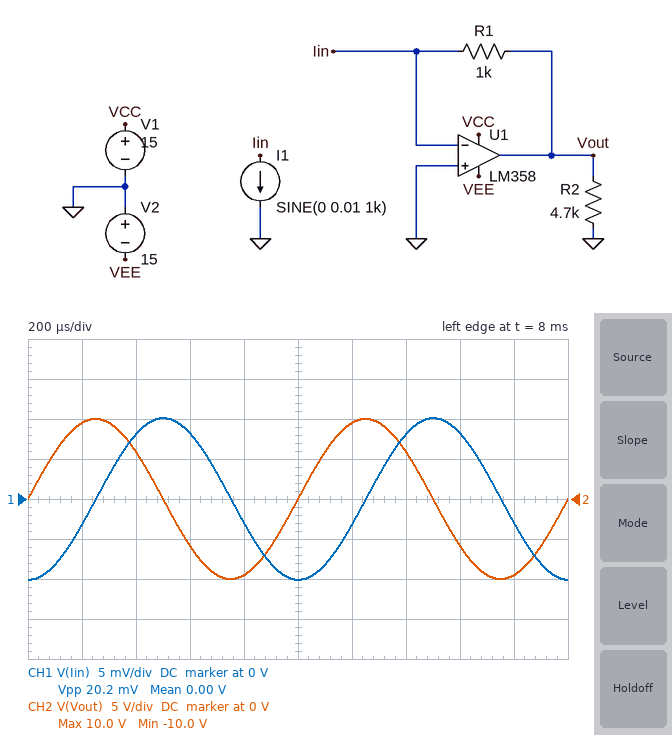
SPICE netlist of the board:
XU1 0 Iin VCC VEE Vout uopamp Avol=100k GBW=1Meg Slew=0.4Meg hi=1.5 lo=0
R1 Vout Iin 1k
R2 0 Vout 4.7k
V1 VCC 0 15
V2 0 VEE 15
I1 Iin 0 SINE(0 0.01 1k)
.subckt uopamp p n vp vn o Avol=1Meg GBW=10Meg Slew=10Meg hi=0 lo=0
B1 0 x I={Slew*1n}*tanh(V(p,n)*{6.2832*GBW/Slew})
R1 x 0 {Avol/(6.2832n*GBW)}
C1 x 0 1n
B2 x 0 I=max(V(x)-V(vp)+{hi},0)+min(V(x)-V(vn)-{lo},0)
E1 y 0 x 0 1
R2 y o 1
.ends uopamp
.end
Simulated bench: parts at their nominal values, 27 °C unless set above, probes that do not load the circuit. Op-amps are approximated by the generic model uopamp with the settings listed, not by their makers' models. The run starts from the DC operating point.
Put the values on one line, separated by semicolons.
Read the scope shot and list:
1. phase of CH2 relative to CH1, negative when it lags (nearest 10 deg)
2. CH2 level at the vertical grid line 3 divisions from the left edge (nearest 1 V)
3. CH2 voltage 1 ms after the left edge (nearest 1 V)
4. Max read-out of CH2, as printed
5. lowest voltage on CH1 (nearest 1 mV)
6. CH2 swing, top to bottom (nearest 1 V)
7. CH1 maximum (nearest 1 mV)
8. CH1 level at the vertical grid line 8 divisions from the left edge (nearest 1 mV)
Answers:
90 deg; -6 V; 0 V; 10.0 V; -10 mV; 20 V; 10 mV; 8 mV
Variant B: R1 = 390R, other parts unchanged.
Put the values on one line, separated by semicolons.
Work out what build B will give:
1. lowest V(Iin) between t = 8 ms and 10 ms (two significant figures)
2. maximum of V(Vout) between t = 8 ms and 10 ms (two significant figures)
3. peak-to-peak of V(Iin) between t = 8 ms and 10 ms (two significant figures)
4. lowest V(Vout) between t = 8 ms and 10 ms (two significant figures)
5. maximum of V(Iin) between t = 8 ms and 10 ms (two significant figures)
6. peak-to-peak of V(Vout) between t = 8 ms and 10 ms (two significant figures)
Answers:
-3.9 mV; 3.9 V; 7.8 mV; -3.9 V; 3.9 mV; 7.8 V
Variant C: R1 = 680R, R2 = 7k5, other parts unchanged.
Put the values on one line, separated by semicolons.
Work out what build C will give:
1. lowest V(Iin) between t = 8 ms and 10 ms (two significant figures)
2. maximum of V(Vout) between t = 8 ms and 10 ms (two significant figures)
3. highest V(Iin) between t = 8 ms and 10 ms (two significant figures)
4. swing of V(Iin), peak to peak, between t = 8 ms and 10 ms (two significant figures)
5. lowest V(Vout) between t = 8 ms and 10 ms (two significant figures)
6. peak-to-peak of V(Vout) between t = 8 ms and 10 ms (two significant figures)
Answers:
-6.8 mV; 6.8 V; 6.8 mV; 14 mV; -6.8 V; 14 V
